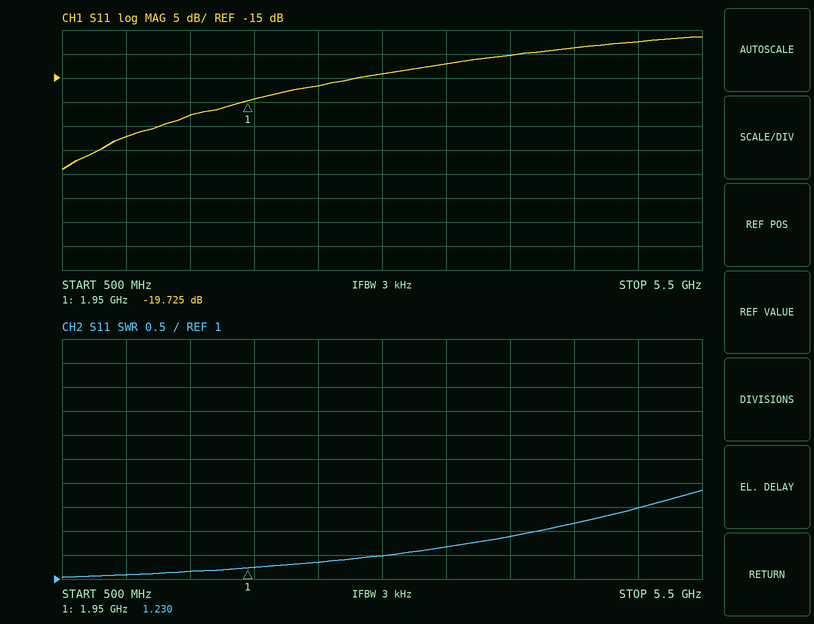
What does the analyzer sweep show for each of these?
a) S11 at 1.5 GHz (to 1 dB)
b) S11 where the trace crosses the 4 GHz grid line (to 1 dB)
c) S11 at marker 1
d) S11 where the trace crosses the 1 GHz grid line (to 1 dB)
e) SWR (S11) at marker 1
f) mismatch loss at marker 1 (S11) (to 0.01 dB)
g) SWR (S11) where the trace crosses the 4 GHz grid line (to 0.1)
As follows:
-23 dB
-10 dB
-19.725 dB
-27 dB
1.230
0.05 dB
1.9
